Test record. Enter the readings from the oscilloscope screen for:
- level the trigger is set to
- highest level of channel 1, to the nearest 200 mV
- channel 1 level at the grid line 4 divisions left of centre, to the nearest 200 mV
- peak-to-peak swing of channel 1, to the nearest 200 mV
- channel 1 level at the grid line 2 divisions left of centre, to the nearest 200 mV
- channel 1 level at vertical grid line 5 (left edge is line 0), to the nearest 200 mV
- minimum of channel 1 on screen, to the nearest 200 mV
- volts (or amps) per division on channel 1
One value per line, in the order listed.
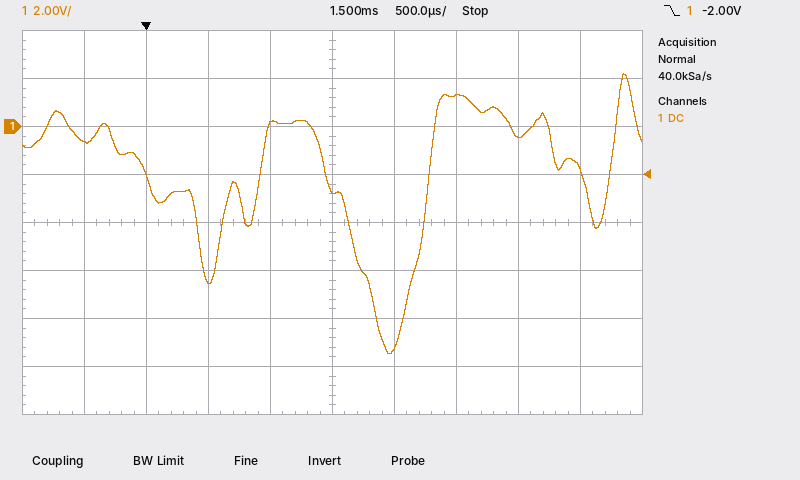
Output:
-2.00 V
2.2 V
-600 mV
11.6 V
-6.4 V
-2.6 V
-9.4 V
2 V
